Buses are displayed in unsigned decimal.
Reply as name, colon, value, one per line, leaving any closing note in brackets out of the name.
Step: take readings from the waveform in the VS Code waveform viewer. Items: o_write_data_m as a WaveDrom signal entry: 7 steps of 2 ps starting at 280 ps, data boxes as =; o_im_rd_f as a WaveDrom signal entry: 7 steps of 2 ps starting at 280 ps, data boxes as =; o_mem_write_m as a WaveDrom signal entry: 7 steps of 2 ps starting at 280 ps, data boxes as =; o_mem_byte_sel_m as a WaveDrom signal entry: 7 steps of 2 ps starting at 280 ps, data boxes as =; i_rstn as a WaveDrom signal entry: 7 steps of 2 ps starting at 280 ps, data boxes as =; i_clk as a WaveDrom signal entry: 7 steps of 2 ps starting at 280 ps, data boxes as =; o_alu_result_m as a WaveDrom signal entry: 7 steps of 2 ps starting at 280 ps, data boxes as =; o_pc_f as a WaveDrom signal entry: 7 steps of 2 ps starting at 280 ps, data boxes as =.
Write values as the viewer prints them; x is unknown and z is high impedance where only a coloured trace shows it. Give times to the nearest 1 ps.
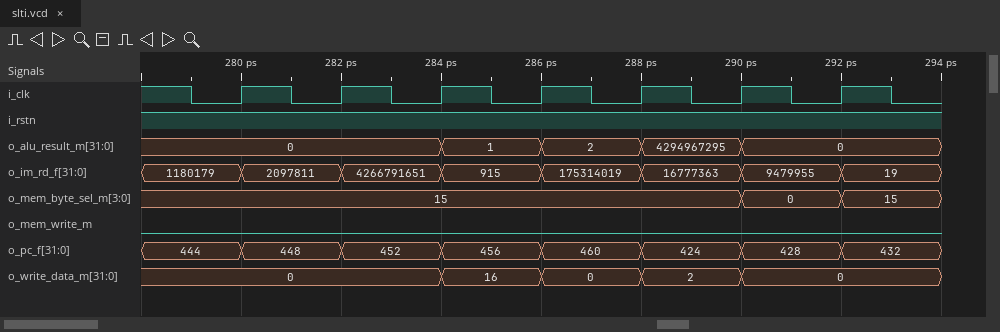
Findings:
o_write_data_m as a WaveDrom signal entry: 7 steps of 2 ps starting at 280 ps, data boxes as =: {name: 'o_write_data_m', wave: '=.====.', data: '0 16 0 2 0'}
o_im_rd_f as a WaveDrom signal entry: 7 steps of 2 ps starting at 280 ps, data boxes as =: {name: 'o_im_rd_f', wave: '=======', data: '2097811 4266791651 915 175314019 16777363 9479955 19'}
o_mem_write_m as a WaveDrom signal entry: 7 steps of 2 ps starting at 280 ps, data boxes as =: {name: 'o_mem_write_m', wave: '0......'}
o_mem_byte_sel_m as a WaveDrom signal entry: 7 steps of 2 ps starting at 280 ps, data boxes as =: {name: 'o_mem_byte_sel_m', wave: '=....==', data: '15 0 15'}
i_rstn as a WaveDrom signal entry: 7 steps of 2 ps starting at 280 ps, data boxes as =: {name: 'i_rstn', wave: '1......'}
i_clk as a WaveDrom signal entry: 7 steps of 2 ps starting at 280 ps, data boxes as =: {name: 'i_clk', wave: 'p......'}
o_alu_result_m as a WaveDrom signal entry: 7 steps of 2 ps starting at 280 ps, data boxes as =: {name: 'o_alu_result_m', wave: '=.====.', data: '0 1 2 4294967295 0'}
o_pc_f as a WaveDrom signal entry: 7 steps of 2 ps starting at 280 ps, data boxes as =: {name: 'o_pc_f', wave: '=======', data: '448 452 456 460 424 428 432'}
